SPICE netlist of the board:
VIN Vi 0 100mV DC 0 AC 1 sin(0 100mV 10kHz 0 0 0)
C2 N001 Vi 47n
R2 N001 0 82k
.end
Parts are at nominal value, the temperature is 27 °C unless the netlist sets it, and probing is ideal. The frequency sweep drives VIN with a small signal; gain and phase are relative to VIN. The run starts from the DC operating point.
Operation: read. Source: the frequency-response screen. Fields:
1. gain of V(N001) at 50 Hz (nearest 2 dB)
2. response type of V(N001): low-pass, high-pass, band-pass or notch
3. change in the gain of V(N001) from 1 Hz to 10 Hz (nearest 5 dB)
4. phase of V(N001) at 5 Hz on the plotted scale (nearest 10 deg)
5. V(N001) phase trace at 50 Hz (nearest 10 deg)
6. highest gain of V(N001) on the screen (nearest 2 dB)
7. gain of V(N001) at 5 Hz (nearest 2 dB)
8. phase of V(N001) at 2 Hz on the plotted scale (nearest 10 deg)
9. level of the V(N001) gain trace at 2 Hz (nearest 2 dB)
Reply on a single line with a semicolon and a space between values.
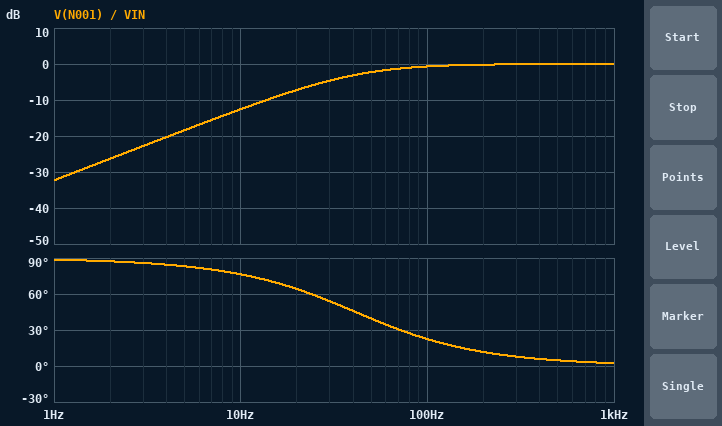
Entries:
-2 dB; high-pass; 20 dB; 80 deg; 40 deg; 0 dB; -18 dB; 90 deg; -26 dB
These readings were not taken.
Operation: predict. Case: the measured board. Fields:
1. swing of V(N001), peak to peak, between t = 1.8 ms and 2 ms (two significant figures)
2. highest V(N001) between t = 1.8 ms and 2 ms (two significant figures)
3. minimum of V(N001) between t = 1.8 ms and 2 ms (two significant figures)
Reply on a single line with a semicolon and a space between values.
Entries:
200 mV; 100 mV; -100 mV
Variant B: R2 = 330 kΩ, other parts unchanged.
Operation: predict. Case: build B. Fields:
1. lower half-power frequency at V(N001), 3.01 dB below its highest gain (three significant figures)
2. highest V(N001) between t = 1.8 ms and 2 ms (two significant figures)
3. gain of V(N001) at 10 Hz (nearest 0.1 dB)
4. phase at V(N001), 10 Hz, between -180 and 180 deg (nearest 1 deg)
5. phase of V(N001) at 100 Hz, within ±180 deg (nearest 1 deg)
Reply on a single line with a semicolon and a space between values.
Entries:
10.3 Hz; 100 mV; -3.1 dB; 46 deg; 6 deg
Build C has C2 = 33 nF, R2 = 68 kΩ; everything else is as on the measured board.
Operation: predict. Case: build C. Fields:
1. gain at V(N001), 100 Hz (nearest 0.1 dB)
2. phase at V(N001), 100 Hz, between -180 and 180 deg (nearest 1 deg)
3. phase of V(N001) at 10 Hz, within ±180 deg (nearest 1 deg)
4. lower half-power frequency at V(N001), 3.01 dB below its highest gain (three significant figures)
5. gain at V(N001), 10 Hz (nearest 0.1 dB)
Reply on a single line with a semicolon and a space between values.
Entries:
-1.8 dB; 35 deg; 82 deg; 70.9 Hz; -17.1 dB
